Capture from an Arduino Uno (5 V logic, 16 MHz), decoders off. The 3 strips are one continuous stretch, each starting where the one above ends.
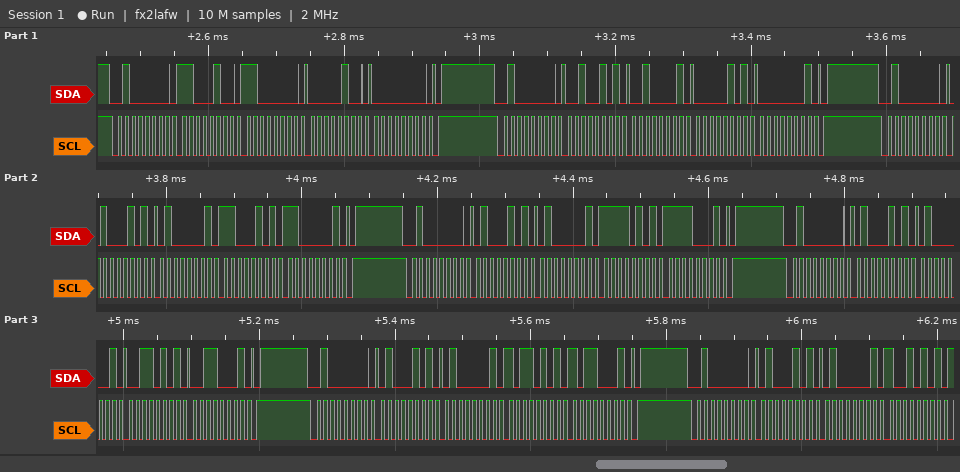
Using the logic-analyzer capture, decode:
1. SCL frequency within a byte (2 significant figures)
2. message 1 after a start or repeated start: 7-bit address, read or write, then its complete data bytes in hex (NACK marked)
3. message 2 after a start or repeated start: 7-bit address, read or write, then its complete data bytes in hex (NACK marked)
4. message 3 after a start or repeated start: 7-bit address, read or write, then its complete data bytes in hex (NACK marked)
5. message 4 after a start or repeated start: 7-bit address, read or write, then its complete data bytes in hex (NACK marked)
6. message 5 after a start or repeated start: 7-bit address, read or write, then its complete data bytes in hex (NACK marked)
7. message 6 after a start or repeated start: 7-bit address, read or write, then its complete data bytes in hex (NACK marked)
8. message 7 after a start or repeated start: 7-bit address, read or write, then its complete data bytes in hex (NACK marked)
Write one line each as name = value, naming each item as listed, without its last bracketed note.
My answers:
SCL frequency within a byte = 100 kHz
message 1 after a start or repeated start: 7-bit address, read or write, then its complete data bytes in hex = 0x20 write: C4 C0 04 00
message 2 after a start or repeated start: 7-bit address, read or write, then its complete data bytes in hex = 0x20 write: 25 21 05 01
message 3 after a start or repeated start: 7-bit address, read or write, then its complete data bytes in hex = 0x20 write: 45 41 C5 C1
message 4 after a start or repeated start: 7-bit address, read or write, then its complete data bytes in hex = 0x20 write: 45 41 F5 F1
message 5 after a start or repeated start: 7-bit address, read or write, then its complete data bytes in hex = 0x20 write: 45 41 35 31
message 6 after a start or repeated start: 7-bit address, read or write, then its complete data bytes in hex = 0x20 write: 45 41 B5 B1
message 7 after a start or repeated start: 7-bit address, read or write, then its complete data bytes in hex = 0x20 write: 45 41 95
